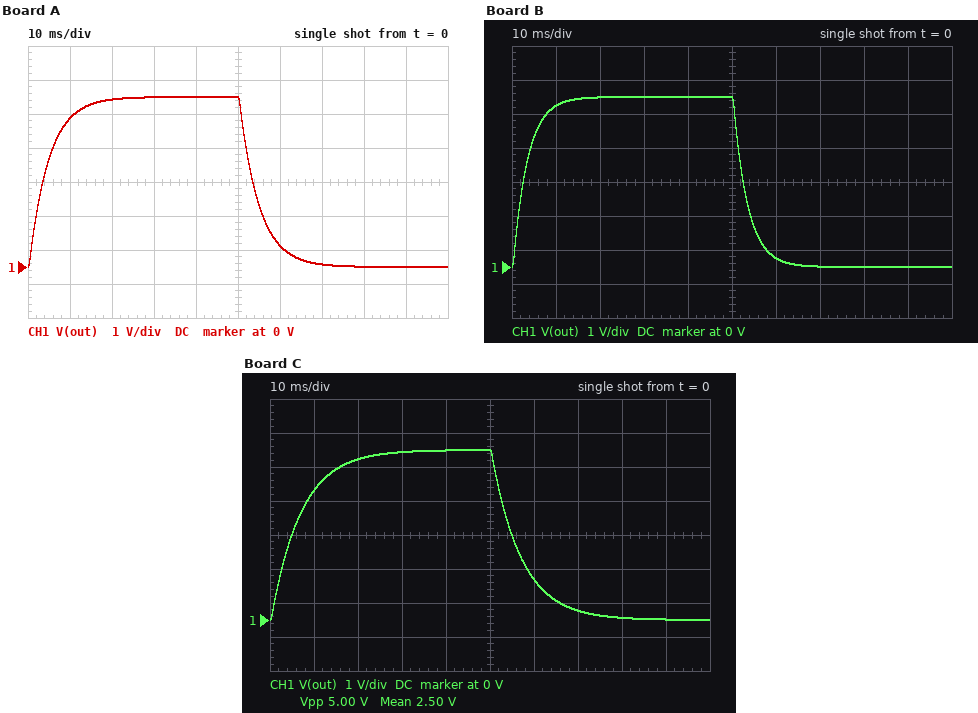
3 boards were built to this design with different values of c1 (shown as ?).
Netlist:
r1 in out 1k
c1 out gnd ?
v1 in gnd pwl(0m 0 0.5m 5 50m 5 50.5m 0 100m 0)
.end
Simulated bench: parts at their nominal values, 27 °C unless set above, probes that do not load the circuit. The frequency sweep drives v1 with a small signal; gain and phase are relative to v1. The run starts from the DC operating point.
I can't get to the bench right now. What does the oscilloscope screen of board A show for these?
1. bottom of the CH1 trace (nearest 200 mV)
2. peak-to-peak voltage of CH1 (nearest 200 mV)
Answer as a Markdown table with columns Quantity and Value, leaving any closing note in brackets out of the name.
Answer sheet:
| Quantity | Value |
|---|---|
| bottom of the CH1 trace | 0 V |
| peak-to-peak voltage of CH1 | 5.0 V |
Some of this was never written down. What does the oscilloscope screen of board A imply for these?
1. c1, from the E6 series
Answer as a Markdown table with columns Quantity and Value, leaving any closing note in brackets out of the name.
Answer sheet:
| Quantity | Value |
|---|---|
| c1, from the E6 series | 4.7 µF |
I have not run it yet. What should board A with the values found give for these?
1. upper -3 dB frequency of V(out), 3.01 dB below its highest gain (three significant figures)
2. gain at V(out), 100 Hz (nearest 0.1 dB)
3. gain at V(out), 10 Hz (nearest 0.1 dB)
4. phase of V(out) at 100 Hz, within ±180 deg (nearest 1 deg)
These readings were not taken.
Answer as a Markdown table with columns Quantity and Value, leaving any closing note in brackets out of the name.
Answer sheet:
| Quantity | Value |
|---|---|
| upper -3 dB frequency of V(out), 3.01 dB below its highest gain | 33.9 Hz |
| gain at V(out), 100 Hz | -9.9 dB |
| gain at V(out), 10 Hz | -0.4 dB |
| phase of V(out) at 100 Hz, within ±180 deg | -71 deg |
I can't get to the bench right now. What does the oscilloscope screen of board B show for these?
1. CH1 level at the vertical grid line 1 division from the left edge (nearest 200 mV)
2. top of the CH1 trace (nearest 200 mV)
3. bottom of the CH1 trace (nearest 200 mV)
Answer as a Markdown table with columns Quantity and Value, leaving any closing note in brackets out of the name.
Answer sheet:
| Quantity | Value |
|---|---|
| CH1 level at the vertical grid line 1 division from the left edge | 4.8 V |
| top of the CH1 trace | 5.0 V |
| bottom of the CH1 trace | 0 V |
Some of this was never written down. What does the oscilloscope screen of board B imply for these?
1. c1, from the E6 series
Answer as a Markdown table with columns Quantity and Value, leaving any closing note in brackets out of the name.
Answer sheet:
| Quantity | Value |
|---|---|
| c1, from the E6 series | 3.3 µF |
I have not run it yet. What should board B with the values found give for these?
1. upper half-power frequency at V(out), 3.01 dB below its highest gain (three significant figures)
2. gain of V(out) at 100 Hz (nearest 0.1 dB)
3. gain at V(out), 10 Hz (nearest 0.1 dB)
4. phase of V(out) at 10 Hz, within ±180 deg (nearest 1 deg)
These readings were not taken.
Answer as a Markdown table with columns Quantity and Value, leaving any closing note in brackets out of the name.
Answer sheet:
| Quantity | Value |
|---|---|
| upper half-power frequency at V(out), 3.01 dB below its highest gain | 48.2 Hz |
| gain of V(out) at 100 Hz | -7.2 dB |
| gain at V(out), 10 Hz | -0.2 dB |
| phase of V(out) at 10 Hz, within ±180 deg | -12 deg |
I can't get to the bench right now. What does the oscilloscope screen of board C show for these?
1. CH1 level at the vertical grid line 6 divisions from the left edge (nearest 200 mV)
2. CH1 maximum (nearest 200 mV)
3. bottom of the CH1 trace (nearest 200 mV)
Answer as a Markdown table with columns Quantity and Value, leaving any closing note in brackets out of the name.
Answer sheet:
| Quantity | Value |
|---|---|
| CH1 level at the vertical grid line 6 divisions from the left edge | 1.2 V |
| CH1 maximum | 5.0 V |
| bottom of the CH1 trace | 0 V |
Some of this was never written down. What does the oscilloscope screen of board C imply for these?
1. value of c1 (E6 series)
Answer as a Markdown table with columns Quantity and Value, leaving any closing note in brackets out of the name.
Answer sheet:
| Quantity | Value |
|---|---|
| value of c1 | 6.8 µF |
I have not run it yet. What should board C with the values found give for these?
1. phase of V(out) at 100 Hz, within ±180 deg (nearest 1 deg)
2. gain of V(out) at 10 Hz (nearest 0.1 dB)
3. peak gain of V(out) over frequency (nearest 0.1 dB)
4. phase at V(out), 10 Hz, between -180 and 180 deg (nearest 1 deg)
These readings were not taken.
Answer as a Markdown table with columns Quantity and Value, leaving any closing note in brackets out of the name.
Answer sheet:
| Quantity | Value |
|---|---|
| phase of V(out) at 100 Hz, within ±180 deg | -77 deg |
| gain of V(out) at 10 Hz | -0.7 dB |
| peak gain of V(out) over frequency | 0 dB |
| phase at V(out), 10 Hz, between -180 and 180 deg | -23 deg |
